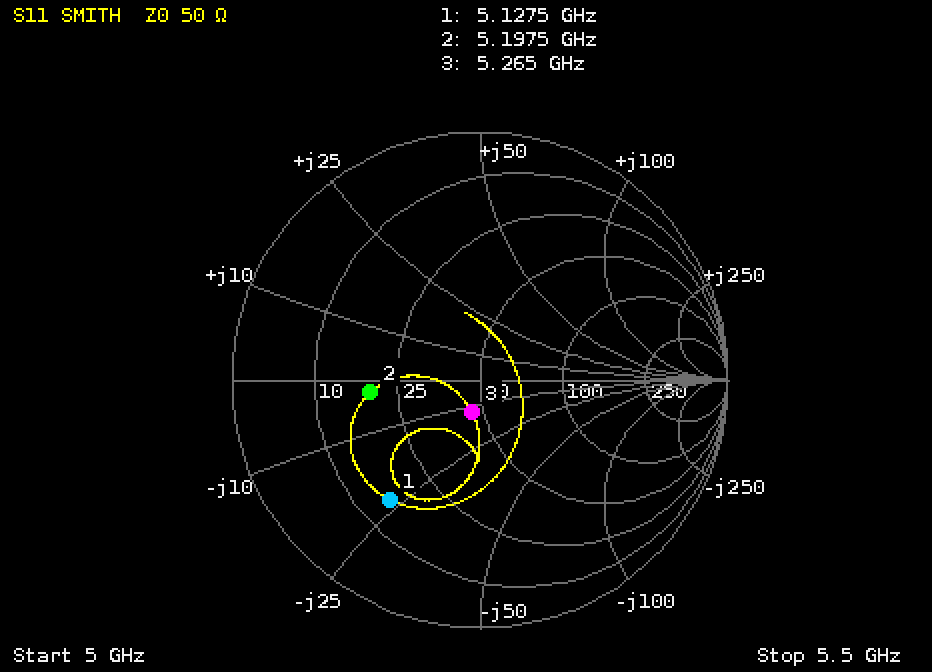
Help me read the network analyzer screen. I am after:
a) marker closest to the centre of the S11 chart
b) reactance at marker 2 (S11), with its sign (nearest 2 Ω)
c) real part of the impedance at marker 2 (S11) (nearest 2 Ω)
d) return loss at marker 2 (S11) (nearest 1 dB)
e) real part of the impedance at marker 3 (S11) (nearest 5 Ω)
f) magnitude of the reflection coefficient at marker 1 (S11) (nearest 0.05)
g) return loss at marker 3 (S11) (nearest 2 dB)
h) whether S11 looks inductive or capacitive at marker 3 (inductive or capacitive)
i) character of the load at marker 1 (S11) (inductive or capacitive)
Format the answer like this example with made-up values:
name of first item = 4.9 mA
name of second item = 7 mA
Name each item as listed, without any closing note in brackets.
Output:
marker closest to the centre of the S11 chart = marker 3
reactance at marker 2 (S11), with its sign = -2 Ω
real part of the impedance at marker 2 (S11) = 20 Ω
return loss at marker 2 (S11) = 7 dB
real part of the impedance at marker 3 (S11) = 45 Ω
magnitude of the reflection coefficient at marker 1 (S11) = 0.60
return loss at marker 3 (S11) = 18 dB
whether S11 looks inductive or capacitive at marker 3 = capacitive
character of the load at marker 1 (S11) = capacitive
